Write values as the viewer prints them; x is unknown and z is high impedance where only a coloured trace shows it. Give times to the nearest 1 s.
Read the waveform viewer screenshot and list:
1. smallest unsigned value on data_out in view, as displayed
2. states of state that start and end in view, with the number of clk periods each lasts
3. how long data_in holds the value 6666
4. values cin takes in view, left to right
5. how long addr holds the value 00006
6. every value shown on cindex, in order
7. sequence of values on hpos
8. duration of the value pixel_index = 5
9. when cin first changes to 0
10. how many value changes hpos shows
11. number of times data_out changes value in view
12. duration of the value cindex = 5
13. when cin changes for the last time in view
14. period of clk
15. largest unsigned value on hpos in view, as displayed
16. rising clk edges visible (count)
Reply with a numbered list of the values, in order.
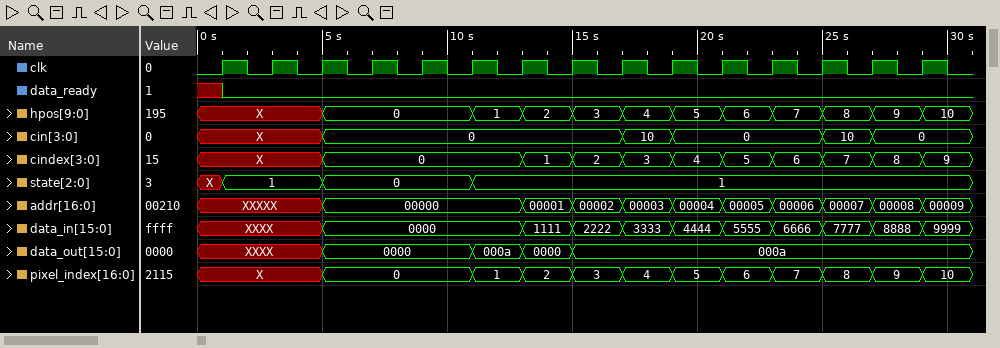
1. 0000
2. 1: 2, 0: 3
3. 2 s
4. X, 0, 10, 0, 10, 0
5. 2 s
6. X, 0, 1, 2, 3, 4, 5, 6, 7, 8, 9
7. X, 0, 1, 2, 3, 4, 5, 6, 7, 8, 9, 10
8. 2 s
9. 5 s
10. 11
11. 4
12. 2 s
13. 27 s
14. 2 s
15. 10
16. 15
